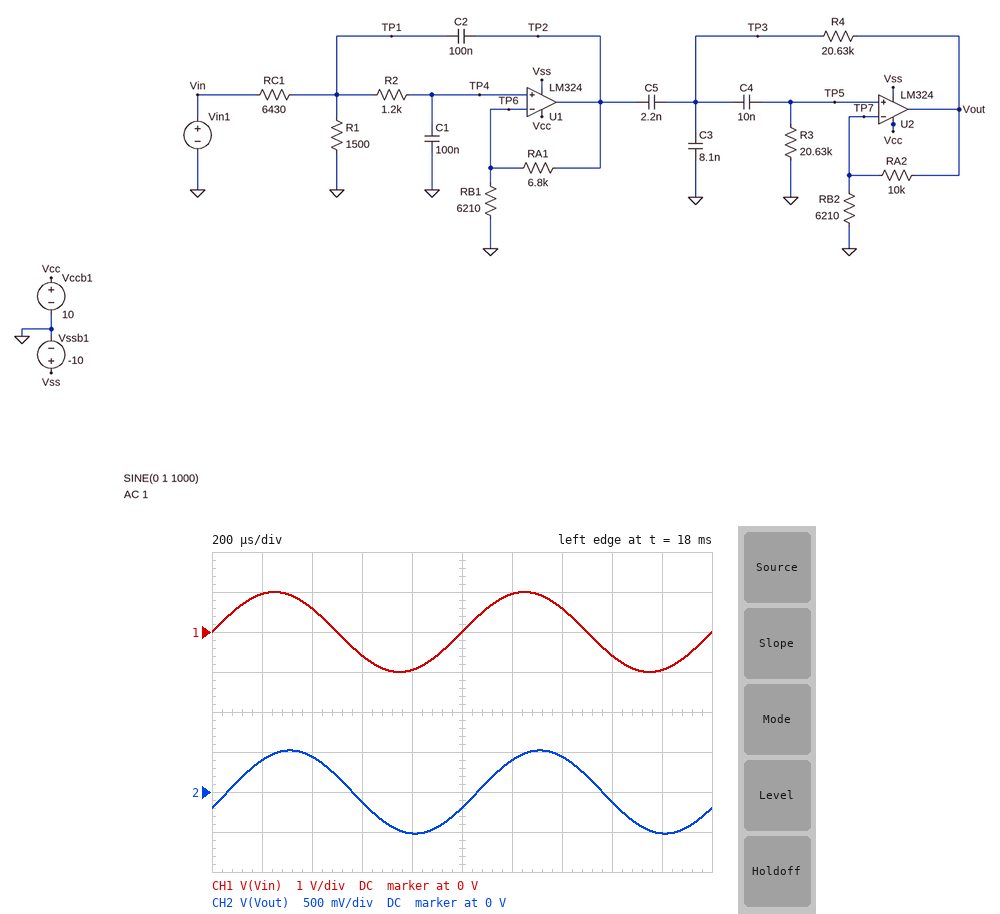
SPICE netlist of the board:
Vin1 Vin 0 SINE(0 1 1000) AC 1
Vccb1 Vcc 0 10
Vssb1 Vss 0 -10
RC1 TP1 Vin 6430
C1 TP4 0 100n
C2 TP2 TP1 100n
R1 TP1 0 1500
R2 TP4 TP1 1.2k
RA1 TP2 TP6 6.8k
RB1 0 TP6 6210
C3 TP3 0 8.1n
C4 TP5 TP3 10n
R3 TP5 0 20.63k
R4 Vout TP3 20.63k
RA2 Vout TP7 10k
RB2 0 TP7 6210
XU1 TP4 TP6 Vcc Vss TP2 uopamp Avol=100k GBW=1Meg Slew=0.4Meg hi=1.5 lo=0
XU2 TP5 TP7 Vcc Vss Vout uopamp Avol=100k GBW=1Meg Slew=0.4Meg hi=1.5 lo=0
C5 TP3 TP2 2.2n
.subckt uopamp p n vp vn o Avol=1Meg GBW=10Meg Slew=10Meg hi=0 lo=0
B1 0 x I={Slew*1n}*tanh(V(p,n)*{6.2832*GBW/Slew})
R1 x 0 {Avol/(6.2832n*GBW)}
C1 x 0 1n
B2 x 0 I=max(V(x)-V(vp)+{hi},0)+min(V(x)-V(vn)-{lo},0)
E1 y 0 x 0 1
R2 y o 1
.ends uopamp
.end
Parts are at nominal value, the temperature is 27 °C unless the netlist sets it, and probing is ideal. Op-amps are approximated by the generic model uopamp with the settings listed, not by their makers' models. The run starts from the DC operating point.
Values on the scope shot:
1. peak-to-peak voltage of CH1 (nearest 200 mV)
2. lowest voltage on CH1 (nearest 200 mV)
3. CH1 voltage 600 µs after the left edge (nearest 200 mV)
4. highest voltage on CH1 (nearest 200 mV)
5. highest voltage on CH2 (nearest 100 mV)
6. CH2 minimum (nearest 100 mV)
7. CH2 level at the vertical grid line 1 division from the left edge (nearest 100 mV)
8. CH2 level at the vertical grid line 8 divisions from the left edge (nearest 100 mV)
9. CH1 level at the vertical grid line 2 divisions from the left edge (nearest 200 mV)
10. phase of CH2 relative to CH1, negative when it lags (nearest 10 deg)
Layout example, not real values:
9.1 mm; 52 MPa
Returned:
2.0 V; -1.0 V; -600 mV; 1.0 V; 500 mV; -500 mV; 400 mV; -100 mV; 600 mV; -20 deg
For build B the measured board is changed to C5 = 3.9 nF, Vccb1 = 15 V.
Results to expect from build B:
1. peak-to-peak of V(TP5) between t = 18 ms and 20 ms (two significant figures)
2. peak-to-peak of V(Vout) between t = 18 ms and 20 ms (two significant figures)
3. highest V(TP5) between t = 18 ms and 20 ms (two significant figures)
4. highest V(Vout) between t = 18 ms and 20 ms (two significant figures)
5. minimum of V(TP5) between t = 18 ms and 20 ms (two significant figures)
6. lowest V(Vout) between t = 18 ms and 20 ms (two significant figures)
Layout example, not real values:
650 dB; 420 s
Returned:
510 mV; 1.3 V; 250 mV; 660 mV; -250 mV; -660 mV
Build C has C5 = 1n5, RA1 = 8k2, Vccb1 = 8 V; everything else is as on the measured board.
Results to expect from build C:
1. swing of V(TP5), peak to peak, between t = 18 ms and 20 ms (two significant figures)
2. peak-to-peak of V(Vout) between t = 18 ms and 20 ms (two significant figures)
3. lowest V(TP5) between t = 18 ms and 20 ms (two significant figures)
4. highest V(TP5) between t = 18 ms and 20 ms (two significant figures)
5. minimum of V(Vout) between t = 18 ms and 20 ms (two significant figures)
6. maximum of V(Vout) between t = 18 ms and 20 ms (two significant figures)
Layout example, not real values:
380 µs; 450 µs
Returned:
440 mV; 1.1 V; -220 mV; 220 mV; -570 mV; 570 mV
